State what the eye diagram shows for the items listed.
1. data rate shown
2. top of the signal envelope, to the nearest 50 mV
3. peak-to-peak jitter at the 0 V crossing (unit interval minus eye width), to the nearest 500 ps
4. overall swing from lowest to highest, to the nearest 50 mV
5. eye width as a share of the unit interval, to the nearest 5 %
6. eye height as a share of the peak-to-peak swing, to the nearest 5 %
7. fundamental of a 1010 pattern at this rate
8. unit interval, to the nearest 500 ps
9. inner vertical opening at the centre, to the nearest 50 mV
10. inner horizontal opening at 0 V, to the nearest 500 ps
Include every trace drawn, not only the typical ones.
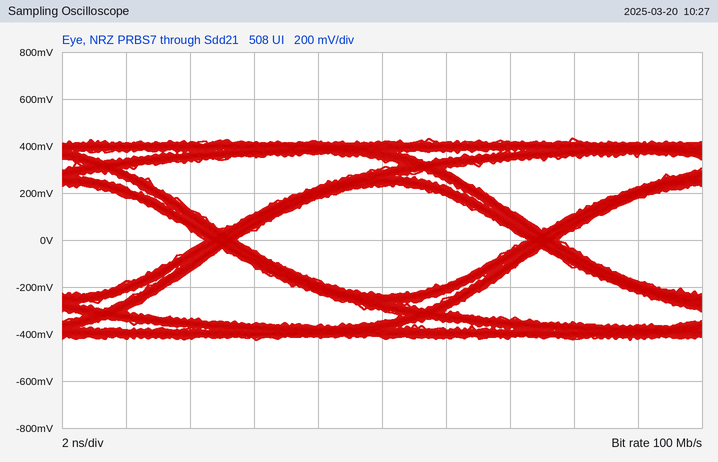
100 Mb/s
450 mV
1.0 ns
850 mV
90 %
55 %
50 MHz
10.0 ns
450 mV
9.0 ns
